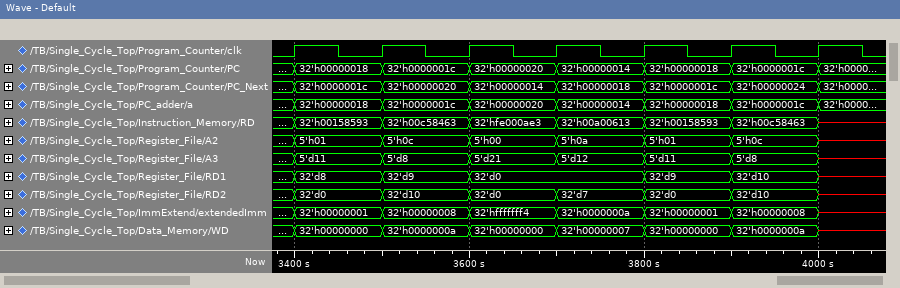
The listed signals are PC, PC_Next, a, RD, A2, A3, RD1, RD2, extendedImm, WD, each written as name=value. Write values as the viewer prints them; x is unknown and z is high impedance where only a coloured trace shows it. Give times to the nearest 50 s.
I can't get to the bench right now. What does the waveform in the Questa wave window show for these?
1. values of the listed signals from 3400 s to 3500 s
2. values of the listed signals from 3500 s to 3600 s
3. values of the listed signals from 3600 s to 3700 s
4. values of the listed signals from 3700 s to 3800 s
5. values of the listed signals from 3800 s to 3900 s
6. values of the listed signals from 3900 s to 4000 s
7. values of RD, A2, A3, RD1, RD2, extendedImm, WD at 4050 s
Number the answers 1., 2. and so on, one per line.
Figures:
1. PC=32'h00000018, PC_Next=32'h0000001c, a=32'h00000018, RD=32'h00158593, A2=5'h01, A3=5'd11, RD1=32'd8, RD2=32'd0, extendedImm=32'h00000001, WD=32'h00000000
2. PC=32'h0000001c, PC_Next=32'h00000020, a=32'h0000001c, RD=32'h00c58463, A2=5'h0c, A3=5'd8, RD1=32'd9, RD2=32'd10, extendedImm=32'h00000008, WD=32'h0000000a
3. PC=32'h00000020, PC_Next=32'h00000014, a=32'h00000020, RD=32'hfe000ae3, A2=5'h00, A3=5'd21, RD1=32'd0, RD2=32'd0, extendedImm=32'hfffffff4, WD=32'h00000000
4. PC=32'h00000014, PC_Next=32'h00000018, a=32'h00000014, RD=32'h00a00613, A2=5'h0a, A3=5'd12, RD1=32'd0, RD2=32'd7, extendedImm=32'h0000000a, WD=32'h00000007
5. PC=32'h00000018, PC_Next=32'h0000001c, a=32'h00000018, RD=32'h00158593, A2=5'h01, A3=5'd11, RD1=32'd9, RD2=32'd0, extendedImm=32'h00000001, WD=32'h00000000
6. PC=32'h0000001c, PC_Next=32'h00000024, a=32'h0000001c, RD=32'h00c58463, A2=5'h0c, A3=5'd8, RD1=32'd10, RD2=32'd10, extendedImm=32'h00000008, WD=32'h0000000a
7. RD=x, A2=x, A3=x, RD1=x, RD2=x, extendedImm=x, WD=x
